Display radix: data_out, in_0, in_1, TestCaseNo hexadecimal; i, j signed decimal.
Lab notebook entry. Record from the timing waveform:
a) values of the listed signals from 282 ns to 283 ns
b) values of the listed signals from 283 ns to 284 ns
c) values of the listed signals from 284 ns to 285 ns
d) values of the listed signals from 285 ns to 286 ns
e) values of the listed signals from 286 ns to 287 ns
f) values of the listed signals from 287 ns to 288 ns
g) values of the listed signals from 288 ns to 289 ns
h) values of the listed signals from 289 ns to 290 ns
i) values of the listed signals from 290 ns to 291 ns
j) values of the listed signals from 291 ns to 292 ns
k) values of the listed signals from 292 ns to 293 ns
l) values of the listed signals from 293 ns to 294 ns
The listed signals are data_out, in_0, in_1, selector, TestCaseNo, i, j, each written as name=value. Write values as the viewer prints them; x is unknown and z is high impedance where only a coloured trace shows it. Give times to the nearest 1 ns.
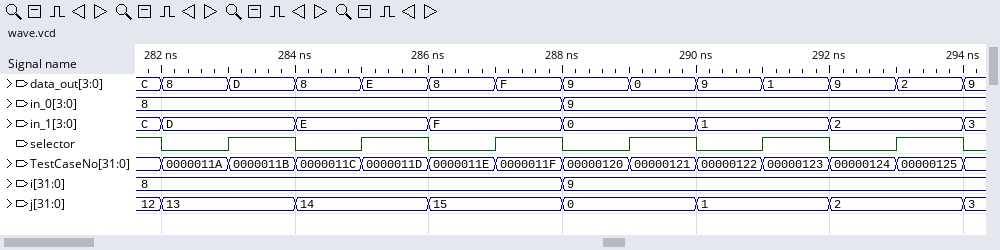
data_out=8, in_0=8, in_1=D, selector=0, TestCaseNo=0000011A, i=8, j=13
data_out=D, in_0=8, in_1=D, selector=1, TestCaseNo=0000011B, i=8, j=13
data_out=8, in_0=8, in_1=E, selector=0, TestCaseNo=0000011C, i=8, j=14
data_out=E, in_0=8, in_1=E, selector=1, TestCaseNo=0000011D, i=8, j=14
data_out=8, in_0=8, in_1=F, selector=0, TestCaseNo=0000011E, i=8, j=15
data_out=F, in_0=8, in_1=F, selector=1, TestCaseNo=0000011F, i=8, j=15
data_out=9, in_0=9, in_1=0, selector=0, TestCaseNo=00000120, i=9, j=0
data_out=0, in_0=9, in_1=0, selector=1, TestCaseNo=00000121, i=9, j=0
data_out=9, in_0=9, in_1=1, selector=0, TestCaseNo=00000122, i=9, j=1
data_out=1, in_0=9, in_1=1, selector=1, TestCaseNo=00000123, i=9, j=1
data_out=9, in_0=9, in_1=2, selector=0, TestCaseNo=00000124, i=9, j=2
data_out=2, in_0=9, in_1=2, selector=1, TestCaseNo=00000125, i=9, j=2
